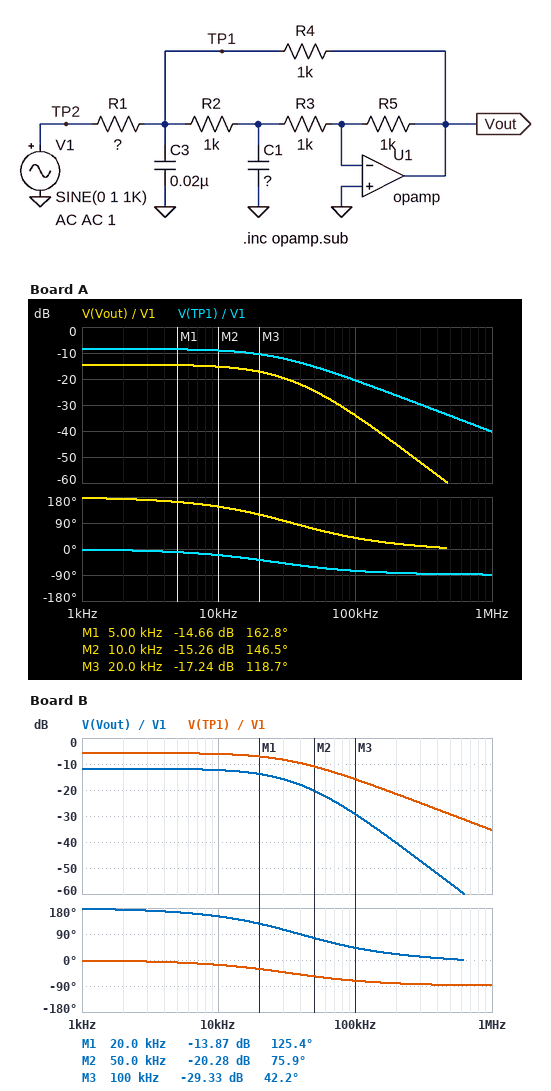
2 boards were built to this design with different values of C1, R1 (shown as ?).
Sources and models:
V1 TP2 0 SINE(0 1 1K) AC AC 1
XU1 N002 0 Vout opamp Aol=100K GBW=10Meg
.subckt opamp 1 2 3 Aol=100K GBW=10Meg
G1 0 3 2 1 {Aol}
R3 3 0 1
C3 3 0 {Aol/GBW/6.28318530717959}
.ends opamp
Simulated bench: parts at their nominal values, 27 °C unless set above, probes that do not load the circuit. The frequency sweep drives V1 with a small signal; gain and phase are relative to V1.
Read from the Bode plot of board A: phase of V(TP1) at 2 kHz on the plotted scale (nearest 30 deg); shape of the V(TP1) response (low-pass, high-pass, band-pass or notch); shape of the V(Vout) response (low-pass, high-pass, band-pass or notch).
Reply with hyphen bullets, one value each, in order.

- 0 deg
- low-pass
- low-pass
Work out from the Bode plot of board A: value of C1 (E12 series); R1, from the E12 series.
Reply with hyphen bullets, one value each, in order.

- 6.8 nF
- 820 Ω
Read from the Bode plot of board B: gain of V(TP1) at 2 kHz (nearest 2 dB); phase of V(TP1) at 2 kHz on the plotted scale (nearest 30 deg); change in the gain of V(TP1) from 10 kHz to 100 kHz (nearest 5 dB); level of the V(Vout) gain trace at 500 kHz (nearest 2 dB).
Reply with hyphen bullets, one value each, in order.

- -6 dB
- 0 deg
- -10 dB
- -56 dB
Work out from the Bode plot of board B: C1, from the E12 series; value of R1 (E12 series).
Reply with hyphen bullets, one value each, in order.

- 6.8 nF
- 470 Ω
